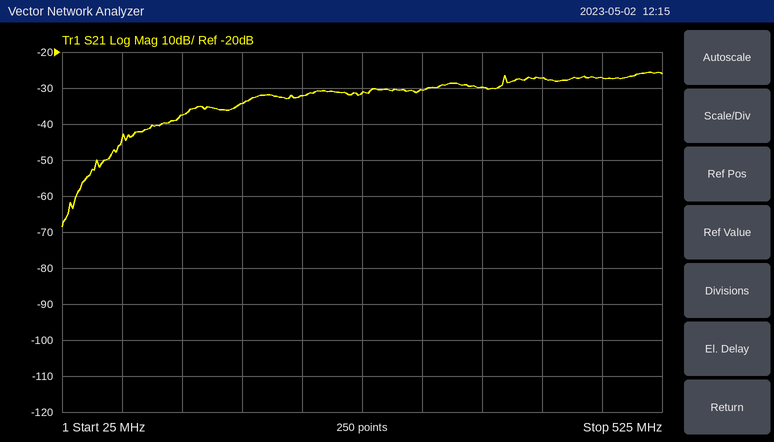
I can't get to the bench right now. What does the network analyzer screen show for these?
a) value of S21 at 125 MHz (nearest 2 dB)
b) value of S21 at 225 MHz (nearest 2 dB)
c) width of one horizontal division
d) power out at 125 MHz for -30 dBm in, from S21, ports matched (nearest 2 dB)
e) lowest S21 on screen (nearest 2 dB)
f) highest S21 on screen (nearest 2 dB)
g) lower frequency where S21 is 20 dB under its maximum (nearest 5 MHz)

-38 dB
-32 dB
50 MHz
-68 dBm
-68 dB
-26 dB
75 MHz
